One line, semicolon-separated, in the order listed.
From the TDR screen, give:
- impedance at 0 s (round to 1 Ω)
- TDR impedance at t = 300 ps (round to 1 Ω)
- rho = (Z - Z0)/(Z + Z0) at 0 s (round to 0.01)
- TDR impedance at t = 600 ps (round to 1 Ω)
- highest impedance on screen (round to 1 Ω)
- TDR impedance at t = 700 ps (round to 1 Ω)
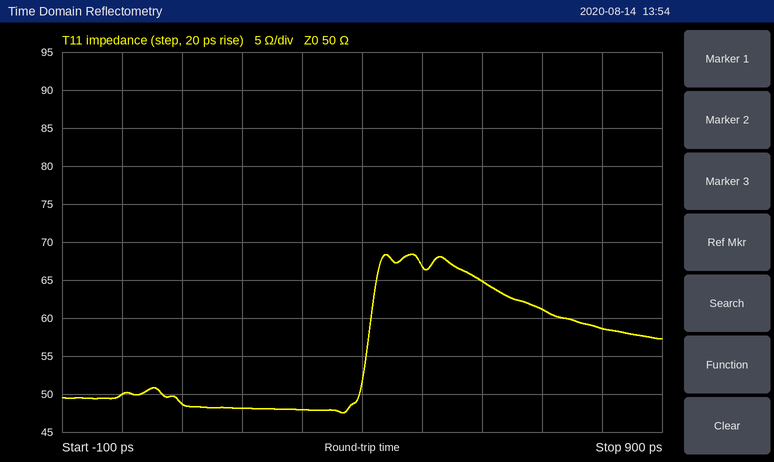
50 Ω; 48 Ω; 0.00; 65 Ω; 68 Ω; 61 Ω
